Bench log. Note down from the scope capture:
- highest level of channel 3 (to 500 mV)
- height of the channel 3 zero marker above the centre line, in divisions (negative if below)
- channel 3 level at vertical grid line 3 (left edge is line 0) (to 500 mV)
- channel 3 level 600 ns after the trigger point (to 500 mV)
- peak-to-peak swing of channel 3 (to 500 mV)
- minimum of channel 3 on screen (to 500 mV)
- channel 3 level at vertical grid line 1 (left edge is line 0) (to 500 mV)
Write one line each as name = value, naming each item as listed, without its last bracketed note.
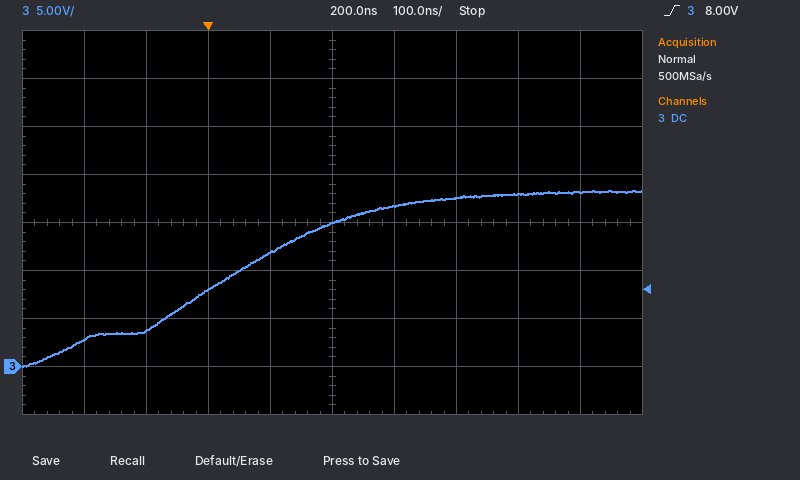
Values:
highest level of channel 3 = 18.5 V
height of the channel 3 zero marker above the centre line, in divisions = -3.0 div
channel 3 level at vertical grid line 3 (left edge is line 0) = 8.0 V
channel 3 level 600 ns after the trigger point = 18.0 V
peak-to-peak swing of channel 3 = 18.5 V
minimum of channel 3 on screen = 0.0 V
channel 3 level at vertical grid line 1 (left edge is line 0) = 3.0 V
